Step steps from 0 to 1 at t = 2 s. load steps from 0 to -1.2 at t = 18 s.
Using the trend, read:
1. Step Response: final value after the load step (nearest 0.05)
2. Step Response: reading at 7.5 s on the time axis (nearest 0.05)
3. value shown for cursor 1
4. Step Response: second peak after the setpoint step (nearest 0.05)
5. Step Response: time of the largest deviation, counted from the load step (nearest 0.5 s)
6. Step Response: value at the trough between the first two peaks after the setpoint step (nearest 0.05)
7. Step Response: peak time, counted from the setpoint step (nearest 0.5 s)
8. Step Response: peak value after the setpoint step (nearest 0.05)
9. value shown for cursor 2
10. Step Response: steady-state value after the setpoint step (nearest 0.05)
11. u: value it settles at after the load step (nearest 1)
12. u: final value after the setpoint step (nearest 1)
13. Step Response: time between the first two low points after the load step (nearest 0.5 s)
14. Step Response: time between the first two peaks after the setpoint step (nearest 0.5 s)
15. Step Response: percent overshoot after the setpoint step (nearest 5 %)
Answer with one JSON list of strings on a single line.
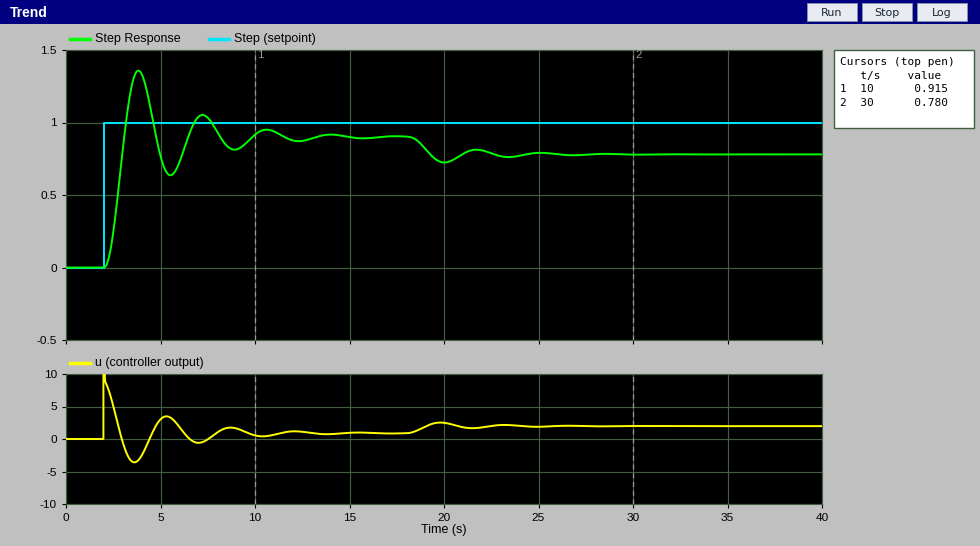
["0.80", "1.05", "0.915", "1.05", "2.0 s", "0.65", "2.0 s", "1.35", "0.780", "0.90", "2", "1", "3.5 s", "3.5 s", "50 %"]
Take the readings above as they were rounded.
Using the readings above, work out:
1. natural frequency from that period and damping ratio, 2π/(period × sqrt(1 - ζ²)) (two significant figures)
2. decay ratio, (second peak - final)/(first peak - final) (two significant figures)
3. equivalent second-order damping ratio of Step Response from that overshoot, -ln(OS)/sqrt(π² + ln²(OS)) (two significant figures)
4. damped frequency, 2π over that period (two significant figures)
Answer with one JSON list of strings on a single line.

["1.8 rad/s", "0.33", "0.22", "1.8 rad/s"]
